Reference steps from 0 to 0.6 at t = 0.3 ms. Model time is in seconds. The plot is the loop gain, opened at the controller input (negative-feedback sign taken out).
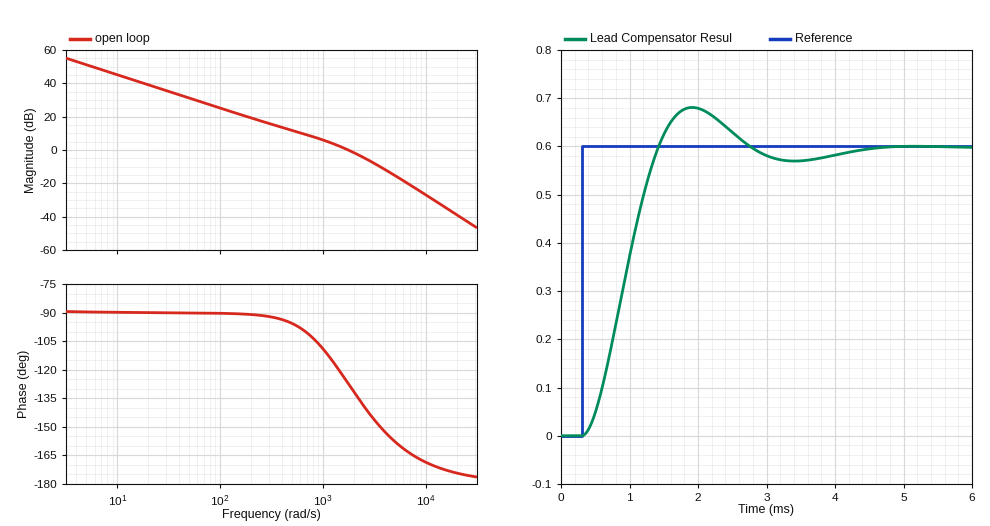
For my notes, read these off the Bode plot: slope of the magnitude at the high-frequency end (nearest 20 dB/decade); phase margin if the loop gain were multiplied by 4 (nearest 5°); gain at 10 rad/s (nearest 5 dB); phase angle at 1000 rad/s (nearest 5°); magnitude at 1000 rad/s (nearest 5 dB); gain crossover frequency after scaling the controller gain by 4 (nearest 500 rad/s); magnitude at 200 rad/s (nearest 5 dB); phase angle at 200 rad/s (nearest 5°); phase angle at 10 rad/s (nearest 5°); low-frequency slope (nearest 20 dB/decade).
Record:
-40 dB/decade
25°
45 dB
-110°
5 dB
4000 rad/s
20 dB
-90°
-90°
-20 dB/decade
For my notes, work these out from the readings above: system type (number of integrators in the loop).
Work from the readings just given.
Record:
1
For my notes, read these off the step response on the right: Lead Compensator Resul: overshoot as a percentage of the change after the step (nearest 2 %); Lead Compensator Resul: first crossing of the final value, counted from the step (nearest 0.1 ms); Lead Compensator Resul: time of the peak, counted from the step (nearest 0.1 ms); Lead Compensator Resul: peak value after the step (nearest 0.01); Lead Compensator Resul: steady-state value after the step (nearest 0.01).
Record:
14 %
1.1 ms
1.6 ms
0.68
0.60
